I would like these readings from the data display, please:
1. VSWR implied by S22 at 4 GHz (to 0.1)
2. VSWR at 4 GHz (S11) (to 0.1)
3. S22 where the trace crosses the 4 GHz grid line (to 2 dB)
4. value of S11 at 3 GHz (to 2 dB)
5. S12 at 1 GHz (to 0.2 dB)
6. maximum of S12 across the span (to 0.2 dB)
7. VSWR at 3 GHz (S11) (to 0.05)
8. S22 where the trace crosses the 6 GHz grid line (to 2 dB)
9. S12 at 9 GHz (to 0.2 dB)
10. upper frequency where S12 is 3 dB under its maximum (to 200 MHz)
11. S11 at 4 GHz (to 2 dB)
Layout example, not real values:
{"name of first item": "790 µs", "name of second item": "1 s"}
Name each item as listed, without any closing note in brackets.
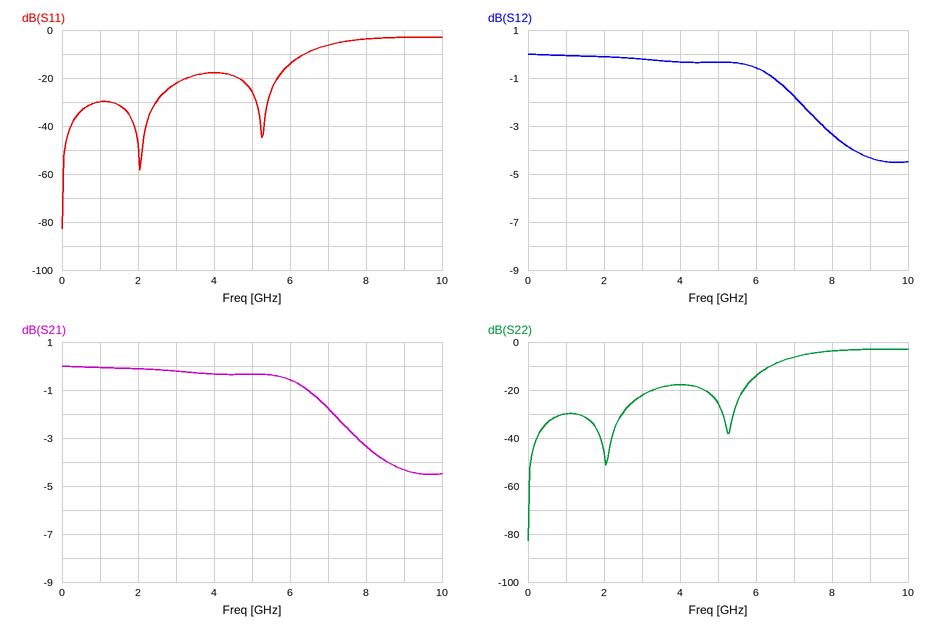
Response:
{"VSWR implied by S22 at 4 GHz": "1.3", "VSWR at 4 GHz (S11)": "1.3", "S22 where the trace crosses the 4 GHz grid line": "-18 dB", "value of S11 at 3 GHz": "-22 dB", "S12 at 1 GHz": "0.0 dB", "maximum of S12 across the span": "0.0 dB", "VSWR at 3 GHz (S11)": "1.15", "S22 where the trace crosses the 6 GHz grid line": "-14 dB", "S12 at 9 GHz": "-4.4 dB", "upper frequency where S12 is 3 dB under its maximum": "7.8 GHz", "S11 at 4 GHz": "-18 dB"}
